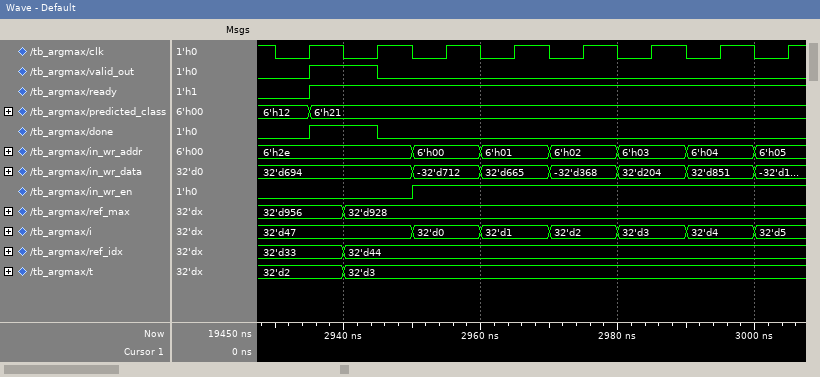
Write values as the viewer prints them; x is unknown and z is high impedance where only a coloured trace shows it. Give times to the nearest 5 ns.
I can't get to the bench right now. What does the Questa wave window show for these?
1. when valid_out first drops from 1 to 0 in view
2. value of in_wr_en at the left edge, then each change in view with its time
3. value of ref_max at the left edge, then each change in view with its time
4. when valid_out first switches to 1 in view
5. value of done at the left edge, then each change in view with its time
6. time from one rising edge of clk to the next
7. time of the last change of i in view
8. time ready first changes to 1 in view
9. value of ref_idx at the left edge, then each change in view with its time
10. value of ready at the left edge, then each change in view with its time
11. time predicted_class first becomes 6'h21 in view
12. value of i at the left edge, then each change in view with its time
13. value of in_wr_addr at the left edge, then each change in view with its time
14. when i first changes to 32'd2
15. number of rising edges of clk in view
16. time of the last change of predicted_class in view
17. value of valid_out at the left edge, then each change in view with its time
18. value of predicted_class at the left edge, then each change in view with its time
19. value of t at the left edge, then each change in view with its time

2945 ns
0, 1 at 2950 ns
32'd956, 32'd928 at 2940 ns
2935 ns
0, 1 at 2935 ns, 0 at 2945 ns
10 ns
3000 ns
2935 ns
32'd33, 32'd44 at 2940 ns
0, 1 at 2935 ns
2935 ns
32'd47, 32'd0 at 2950 ns, 32'd1 at 2960 ns, 32'd2 at 2970 ns, 32'd3 at 2980 ns, 32'd4 at 2990 ns, 32'd5 at 3000 ns
6'h2e, 6'h00 at 2950 ns, 6'h01 at 2960 ns, 6'h02 at 2970 ns, 6'h03 at 2980 ns, 6'h04 at 2990 ns, 6'h05 at 3000 ns
2970 ns
8
2935 ns
0, 1 at 2935 ns, 0 at 2945 ns
6'h12, 6'h21 at 2935 ns
32'd2, 32'd3 at 2940 ns
